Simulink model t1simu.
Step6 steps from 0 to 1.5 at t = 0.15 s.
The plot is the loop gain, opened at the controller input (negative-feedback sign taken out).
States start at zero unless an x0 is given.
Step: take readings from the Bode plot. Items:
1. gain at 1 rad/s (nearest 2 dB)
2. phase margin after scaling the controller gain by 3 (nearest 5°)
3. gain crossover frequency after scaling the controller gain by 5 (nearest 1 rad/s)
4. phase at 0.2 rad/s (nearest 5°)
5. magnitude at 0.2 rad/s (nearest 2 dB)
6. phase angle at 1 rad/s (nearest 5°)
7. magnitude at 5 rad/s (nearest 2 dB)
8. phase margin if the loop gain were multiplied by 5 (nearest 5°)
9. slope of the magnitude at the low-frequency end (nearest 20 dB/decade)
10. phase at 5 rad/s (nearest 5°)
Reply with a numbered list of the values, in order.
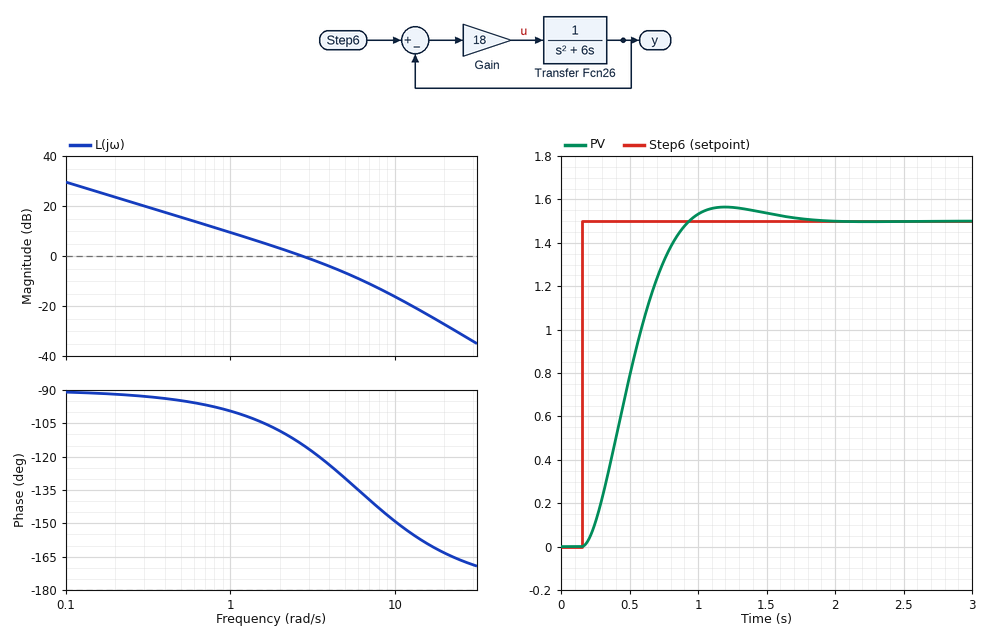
1. 10 dB
2. 45°
3. 9 rad/s
4. -90°
5. 24 dB
6. -100°
7. -6 dB
8. 35°
9. -20 dB/decade
10. -130°
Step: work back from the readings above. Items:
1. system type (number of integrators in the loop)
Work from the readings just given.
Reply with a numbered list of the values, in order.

1. 1
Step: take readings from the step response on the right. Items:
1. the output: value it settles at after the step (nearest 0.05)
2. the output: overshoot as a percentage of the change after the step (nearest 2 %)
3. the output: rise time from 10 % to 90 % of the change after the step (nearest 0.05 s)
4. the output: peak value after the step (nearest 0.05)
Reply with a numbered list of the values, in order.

1. 1.50
2. 4 %
3. 0.50 s
4. 1.55
